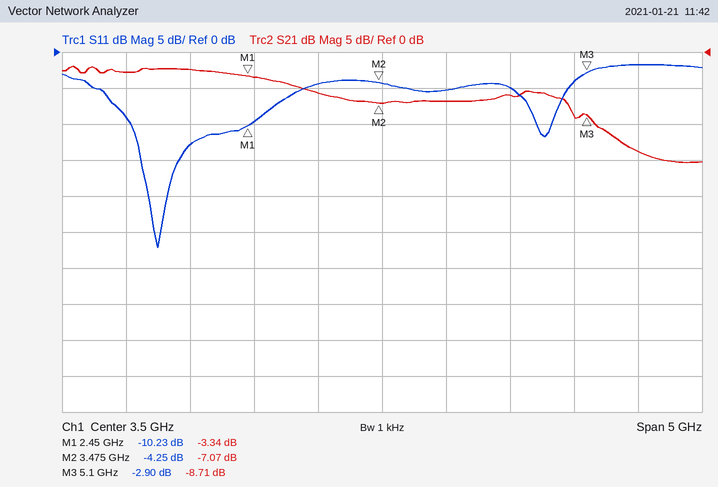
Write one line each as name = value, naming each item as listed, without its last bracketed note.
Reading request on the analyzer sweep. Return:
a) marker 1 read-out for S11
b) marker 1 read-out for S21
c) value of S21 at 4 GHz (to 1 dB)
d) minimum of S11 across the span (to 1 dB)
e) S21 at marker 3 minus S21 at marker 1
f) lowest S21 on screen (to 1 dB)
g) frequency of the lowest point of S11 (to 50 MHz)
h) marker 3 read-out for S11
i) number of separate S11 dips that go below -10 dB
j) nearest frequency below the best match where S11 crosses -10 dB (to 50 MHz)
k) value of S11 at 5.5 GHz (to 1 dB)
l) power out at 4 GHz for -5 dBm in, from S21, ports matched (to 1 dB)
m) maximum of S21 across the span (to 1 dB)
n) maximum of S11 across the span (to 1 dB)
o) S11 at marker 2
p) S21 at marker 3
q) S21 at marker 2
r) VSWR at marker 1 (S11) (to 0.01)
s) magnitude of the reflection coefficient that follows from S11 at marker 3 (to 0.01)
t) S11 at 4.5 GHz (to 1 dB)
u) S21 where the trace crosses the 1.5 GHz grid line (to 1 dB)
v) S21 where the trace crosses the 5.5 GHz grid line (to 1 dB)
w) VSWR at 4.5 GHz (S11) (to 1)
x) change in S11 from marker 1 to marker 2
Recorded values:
marker 1 read-out for S11 = -10.23 dB
marker 1 read-out for S21 = -3.34 dB
value of S21 at 4 GHz = -7 dB
minimum of S11 across the span = -27 dB
S21 at marker 3 minus S21 at marker 1 = -5.37 dB
lowest S21 on screen = -15 dB
frequency of the lowest point of S11 = 1.75 GHz
marker 3 read-out for S11 = -2.90 dB
number of separate S11 dips that go below -10 dB = 2
nearest frequency below the best match where S11 crosses -10 dB = 1.55 GHz
value of S11 at 5.5 GHz = -2 dB
power out at 4 GHz for -5 dBm in, from S21, ports matched = -12 dBm
maximum of S21 across the span = -2 dB
maximum of S11 across the span = -2 dB
S11 at marker 2 = -4.25 dB
S21 at marker 3 = -8.71 dB
S21 at marker 2 = -7.07 dB
VSWR at marker 1 (S11) = 1.89
magnitude of the reflection coefficient that follows from S11 at marker 3 = 0.72
S11 at 4.5 GHz = -5 dB
S21 where the trace crosses the 1.5 GHz grid line = -3 dB
S21 where the trace crosses the 5.5 GHz grid line = -14 dB
VSWR at 4.5 GHz (S11) = 4
change in S11 from marker 1 to marker 2 = 5.98 dB
